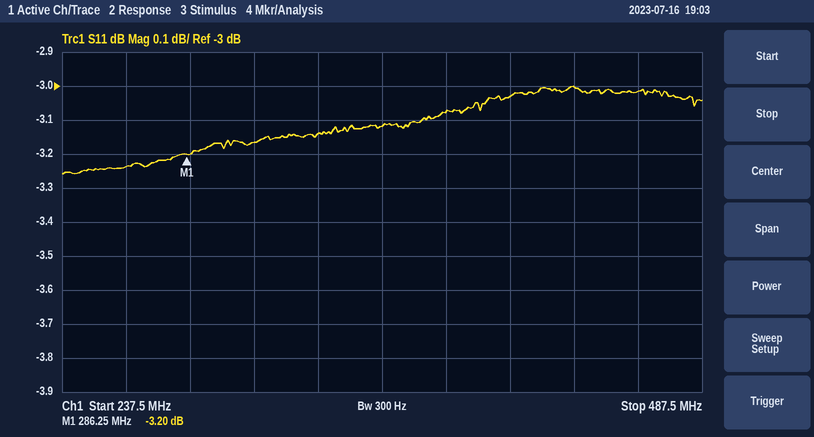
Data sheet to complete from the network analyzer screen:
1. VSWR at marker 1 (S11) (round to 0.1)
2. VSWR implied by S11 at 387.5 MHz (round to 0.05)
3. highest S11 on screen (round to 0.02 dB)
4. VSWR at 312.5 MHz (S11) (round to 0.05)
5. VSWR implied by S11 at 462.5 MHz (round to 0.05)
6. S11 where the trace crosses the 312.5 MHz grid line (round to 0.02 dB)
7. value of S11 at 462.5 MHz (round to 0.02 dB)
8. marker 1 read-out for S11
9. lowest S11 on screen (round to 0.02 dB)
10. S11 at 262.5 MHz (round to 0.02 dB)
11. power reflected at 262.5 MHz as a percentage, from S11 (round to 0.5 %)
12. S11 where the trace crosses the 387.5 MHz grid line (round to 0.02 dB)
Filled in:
5.5
5.70
-3.00 dB
5.55
5.80
-3.16 dB
-3.02 dB
-3.20 dB
-3.26 dB
-3.24 dB
47.5 %
-3.08 dB
